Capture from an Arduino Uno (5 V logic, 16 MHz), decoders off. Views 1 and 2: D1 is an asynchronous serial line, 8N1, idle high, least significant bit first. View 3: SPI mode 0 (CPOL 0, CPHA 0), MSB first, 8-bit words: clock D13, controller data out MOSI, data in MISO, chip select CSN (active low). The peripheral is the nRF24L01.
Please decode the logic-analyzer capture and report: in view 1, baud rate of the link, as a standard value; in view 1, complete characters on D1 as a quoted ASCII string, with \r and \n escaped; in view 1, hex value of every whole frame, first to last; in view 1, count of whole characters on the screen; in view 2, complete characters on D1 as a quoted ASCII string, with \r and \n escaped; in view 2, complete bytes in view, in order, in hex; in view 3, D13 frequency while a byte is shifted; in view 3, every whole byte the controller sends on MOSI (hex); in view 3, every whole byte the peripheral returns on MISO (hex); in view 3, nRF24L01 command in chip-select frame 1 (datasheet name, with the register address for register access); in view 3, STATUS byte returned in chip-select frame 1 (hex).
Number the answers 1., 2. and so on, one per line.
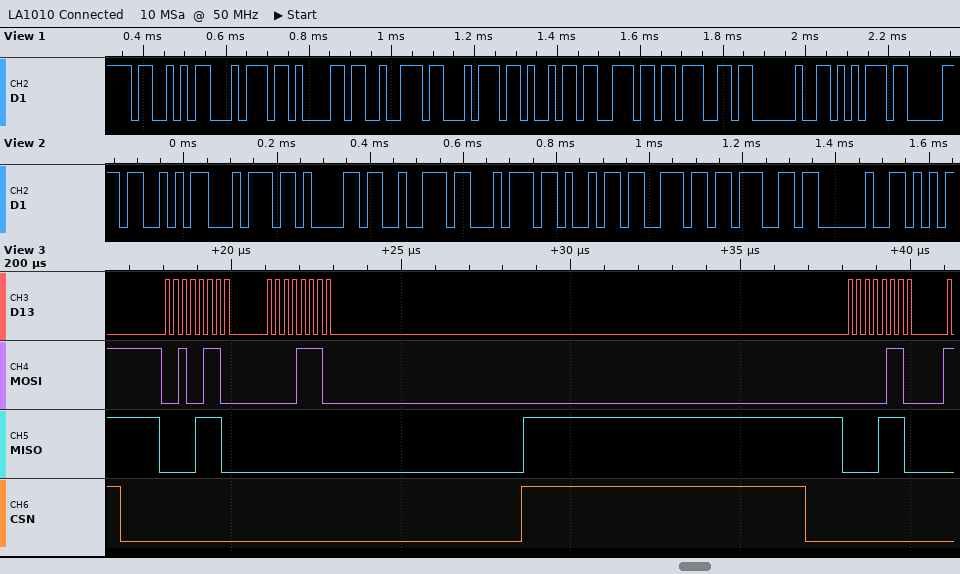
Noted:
1. 57600 baud
2. "Starting u"
3. 53 74 61 72 74 69 6E 67 20 75
4. 10
5. "Starting "
6. 53 74 61 72 74 69 6E 67 20
7. 4 MHz
8. 26 0E 06
9. 0E 00 0E
10. W_REGISTER 0x06
11. 0x0E
